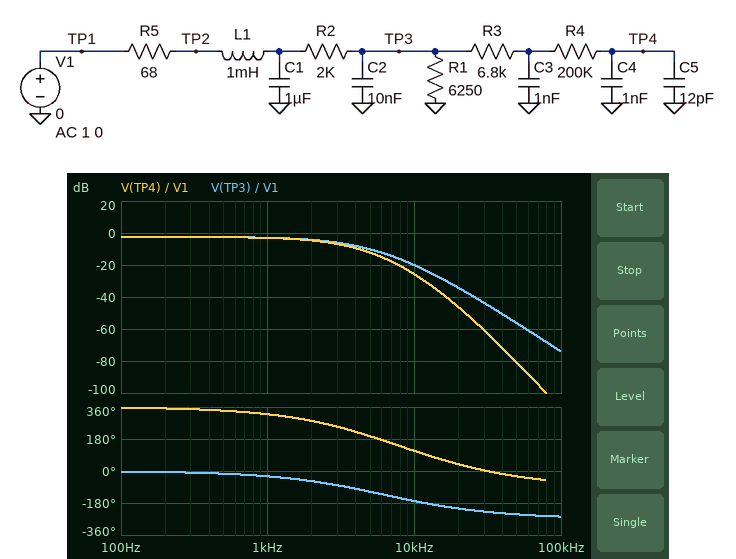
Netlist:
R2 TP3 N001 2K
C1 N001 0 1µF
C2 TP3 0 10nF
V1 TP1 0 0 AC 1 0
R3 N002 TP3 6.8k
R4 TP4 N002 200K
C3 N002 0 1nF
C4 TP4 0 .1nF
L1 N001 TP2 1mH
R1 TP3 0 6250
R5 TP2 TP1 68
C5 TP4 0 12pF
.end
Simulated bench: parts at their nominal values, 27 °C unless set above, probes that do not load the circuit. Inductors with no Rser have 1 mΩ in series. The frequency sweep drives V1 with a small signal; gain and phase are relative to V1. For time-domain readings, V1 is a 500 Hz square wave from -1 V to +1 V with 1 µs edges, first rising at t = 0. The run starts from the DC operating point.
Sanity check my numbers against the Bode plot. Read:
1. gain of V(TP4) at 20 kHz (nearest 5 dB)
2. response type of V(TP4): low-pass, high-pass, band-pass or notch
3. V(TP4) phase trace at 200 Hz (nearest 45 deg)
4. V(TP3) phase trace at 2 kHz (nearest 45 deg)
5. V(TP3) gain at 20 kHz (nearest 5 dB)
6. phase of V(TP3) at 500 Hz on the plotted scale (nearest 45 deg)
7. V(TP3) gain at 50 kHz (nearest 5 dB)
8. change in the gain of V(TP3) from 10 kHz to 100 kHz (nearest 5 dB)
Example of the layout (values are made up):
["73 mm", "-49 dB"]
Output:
["-45 dB", "low-pass", "360 deg", "-45 deg", "-35 dB", "0 deg", "-55 dB", "-55 dB"]
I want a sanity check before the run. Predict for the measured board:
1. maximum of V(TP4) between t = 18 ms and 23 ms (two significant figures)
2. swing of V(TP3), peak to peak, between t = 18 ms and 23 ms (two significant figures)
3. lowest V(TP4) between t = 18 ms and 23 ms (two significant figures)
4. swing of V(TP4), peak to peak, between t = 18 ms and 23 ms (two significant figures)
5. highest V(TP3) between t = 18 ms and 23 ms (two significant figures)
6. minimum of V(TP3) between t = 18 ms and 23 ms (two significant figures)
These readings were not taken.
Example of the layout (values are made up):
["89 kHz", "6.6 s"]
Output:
["750 mV", "1.5 V", "-750 mV", "1.5 V", "750 mV", "-750 mV"]
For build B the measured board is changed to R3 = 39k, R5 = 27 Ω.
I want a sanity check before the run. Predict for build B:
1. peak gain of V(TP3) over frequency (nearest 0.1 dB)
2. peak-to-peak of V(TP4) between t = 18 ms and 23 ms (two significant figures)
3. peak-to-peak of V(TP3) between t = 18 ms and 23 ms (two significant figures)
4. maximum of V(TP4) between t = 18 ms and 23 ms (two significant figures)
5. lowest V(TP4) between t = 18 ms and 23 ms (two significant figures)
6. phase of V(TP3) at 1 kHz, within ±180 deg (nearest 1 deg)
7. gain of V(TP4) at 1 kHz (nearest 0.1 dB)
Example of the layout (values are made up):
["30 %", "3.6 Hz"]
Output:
["-1.0 dB", "1.6 V", "2.1 V", "780 mV", "-780 mV", "-16 deg", "-2.7 dB"]
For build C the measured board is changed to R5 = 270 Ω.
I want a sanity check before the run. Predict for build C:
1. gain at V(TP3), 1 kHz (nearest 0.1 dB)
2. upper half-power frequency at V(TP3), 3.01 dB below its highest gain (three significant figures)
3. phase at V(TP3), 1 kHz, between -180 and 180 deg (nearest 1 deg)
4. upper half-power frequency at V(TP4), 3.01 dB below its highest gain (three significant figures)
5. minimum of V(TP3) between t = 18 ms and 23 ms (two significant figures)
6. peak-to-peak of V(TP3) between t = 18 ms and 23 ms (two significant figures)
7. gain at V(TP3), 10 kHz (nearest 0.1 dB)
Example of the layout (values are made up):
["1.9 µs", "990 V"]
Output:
["-8.4 dB", "610 Hz", "-66 deg", "605 Hz", "-700 mV", "1.4 V", "-30.5 dB"]
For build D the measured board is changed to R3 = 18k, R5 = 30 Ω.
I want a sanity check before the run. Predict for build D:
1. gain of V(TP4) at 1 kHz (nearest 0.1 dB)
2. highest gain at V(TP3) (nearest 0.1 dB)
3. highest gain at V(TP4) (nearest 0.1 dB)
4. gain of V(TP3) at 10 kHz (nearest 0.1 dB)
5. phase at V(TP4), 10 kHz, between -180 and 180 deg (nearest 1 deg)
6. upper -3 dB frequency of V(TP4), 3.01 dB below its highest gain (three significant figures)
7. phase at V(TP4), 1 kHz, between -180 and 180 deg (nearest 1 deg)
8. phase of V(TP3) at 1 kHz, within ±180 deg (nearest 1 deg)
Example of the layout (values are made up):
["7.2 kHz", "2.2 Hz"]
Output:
["-2.5 dB", "-1.6 dB", "-2.4 dB", "-16.5 dB", "67 deg", "4.65 kHz", "-32 deg", "-17 deg"]
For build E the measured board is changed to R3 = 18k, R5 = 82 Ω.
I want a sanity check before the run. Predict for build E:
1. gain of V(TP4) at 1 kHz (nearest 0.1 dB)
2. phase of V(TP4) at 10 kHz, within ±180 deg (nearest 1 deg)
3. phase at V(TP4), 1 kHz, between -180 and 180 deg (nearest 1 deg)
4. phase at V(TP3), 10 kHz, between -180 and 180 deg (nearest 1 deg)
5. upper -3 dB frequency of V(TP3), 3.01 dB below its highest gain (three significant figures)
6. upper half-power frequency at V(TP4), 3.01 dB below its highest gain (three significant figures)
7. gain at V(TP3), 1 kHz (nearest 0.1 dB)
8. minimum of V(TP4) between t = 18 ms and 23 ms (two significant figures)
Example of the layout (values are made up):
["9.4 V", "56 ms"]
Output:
["-3.5 dB", "95 deg", "-49 deg", "-163 deg", "2.14 kHz", "1.87 kHz", "-3.3 dB", "-750 mV"]
